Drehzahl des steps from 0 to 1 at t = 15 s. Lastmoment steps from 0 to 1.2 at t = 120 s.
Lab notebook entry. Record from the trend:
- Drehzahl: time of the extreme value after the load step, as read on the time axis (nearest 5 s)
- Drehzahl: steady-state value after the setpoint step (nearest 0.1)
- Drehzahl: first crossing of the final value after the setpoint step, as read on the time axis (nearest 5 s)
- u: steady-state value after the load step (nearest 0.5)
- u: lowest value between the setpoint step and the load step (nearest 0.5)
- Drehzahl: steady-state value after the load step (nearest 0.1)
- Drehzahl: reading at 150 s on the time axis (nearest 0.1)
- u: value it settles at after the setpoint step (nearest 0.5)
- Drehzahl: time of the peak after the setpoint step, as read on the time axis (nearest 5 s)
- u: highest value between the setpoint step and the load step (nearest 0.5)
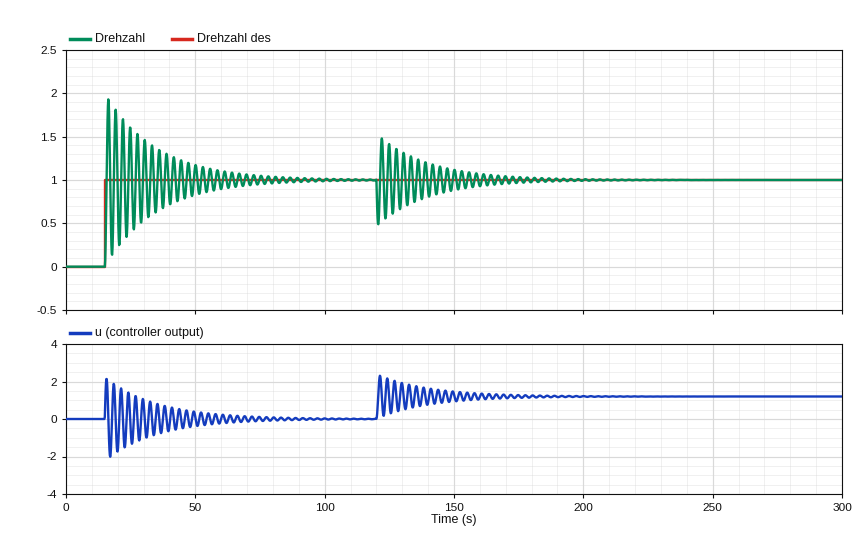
120 s
1.0
15 s
1.0
-2.0
1.0
1.1
0.0
15 s
2.0
